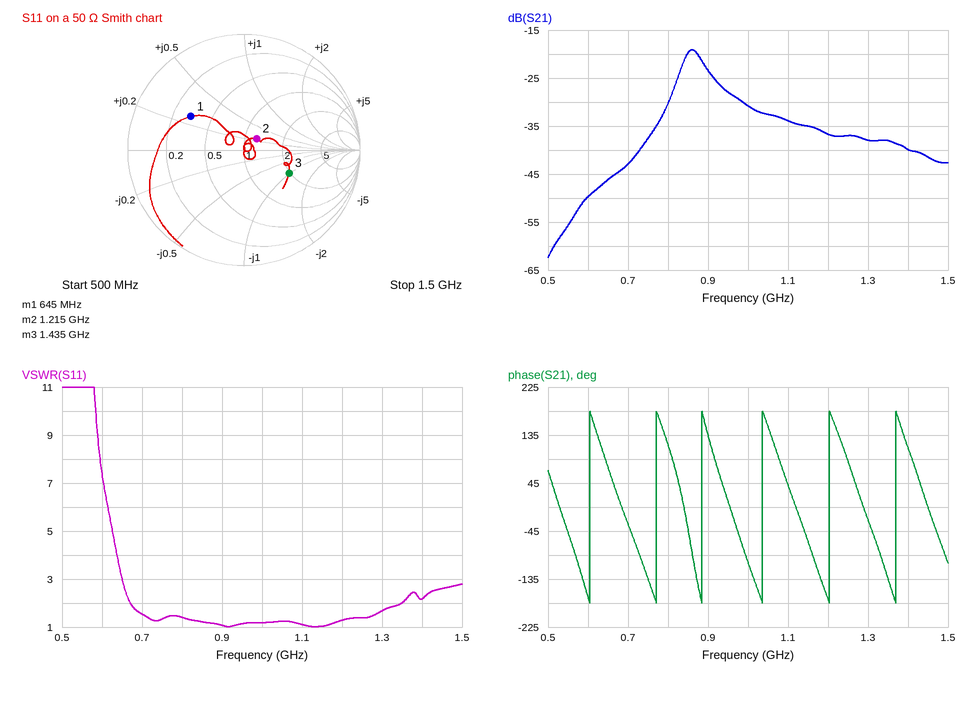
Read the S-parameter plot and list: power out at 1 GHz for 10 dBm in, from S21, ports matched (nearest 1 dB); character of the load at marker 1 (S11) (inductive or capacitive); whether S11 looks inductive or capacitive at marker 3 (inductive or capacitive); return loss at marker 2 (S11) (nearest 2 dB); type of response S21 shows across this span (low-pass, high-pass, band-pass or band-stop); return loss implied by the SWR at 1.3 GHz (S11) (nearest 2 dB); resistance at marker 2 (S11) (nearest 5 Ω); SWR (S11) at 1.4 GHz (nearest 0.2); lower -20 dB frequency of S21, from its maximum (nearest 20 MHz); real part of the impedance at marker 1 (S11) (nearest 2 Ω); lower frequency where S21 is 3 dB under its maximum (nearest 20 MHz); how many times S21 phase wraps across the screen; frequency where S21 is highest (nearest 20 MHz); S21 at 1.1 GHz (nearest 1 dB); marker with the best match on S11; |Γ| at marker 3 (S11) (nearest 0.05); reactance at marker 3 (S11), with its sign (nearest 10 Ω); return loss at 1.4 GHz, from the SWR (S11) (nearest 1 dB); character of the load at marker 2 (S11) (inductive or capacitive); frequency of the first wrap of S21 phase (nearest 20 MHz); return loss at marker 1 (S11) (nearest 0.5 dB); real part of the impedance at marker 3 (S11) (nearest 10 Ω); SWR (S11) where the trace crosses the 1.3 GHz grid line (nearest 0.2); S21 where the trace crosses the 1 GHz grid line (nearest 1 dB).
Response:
-21 dBm
inductive
capacitive
16 dB
band-pass
12 dB
60 Ω
2.2
740 MHz
16 Ω
840 MHz
6
860 MHz
-34 dB
marker 2
0.45
-50 Ω
9 dB
inductive
600 MHz
5.5 dB
100 Ω
1.6
-31 dB
